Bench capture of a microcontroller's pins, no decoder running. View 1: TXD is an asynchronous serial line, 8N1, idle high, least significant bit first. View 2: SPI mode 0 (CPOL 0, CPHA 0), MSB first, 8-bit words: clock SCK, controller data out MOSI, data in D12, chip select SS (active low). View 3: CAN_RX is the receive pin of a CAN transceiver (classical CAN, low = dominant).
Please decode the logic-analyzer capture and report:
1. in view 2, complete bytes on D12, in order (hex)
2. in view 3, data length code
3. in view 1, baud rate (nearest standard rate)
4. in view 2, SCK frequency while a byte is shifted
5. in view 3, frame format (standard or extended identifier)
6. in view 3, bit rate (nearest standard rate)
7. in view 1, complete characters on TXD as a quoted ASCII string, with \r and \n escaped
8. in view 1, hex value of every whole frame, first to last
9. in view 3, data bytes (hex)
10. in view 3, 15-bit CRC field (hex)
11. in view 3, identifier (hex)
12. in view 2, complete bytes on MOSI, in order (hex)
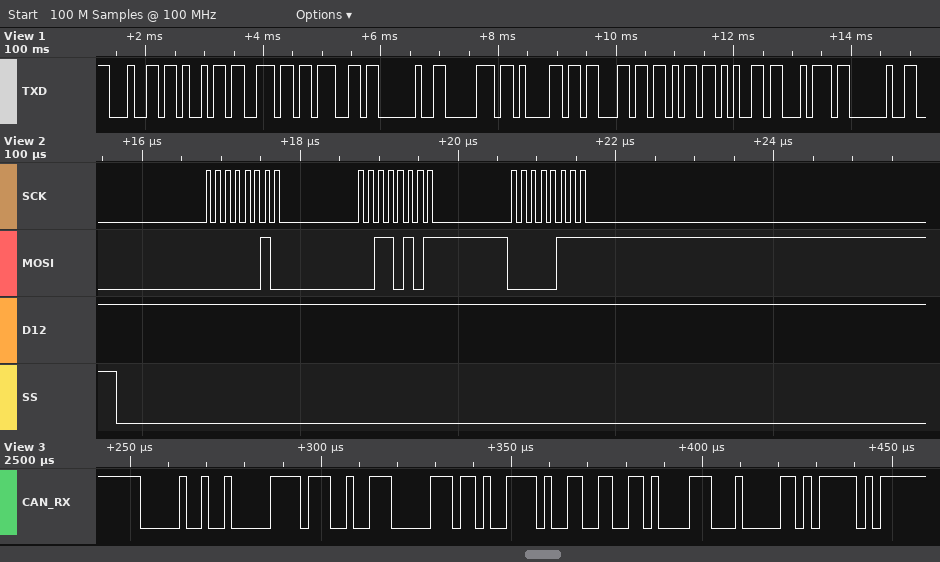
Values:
FF FF FF
7
9600 baud
8 MHz
standard
500 kbit/s
"ding packet "
0x64 0x69 0x6E 0x67 0x20 0x70 0x61 0x63 0x6B 0x65 0x74 0x20
72 70 6D 3D 33 34 38
0x415F
0x012
02 35 07
